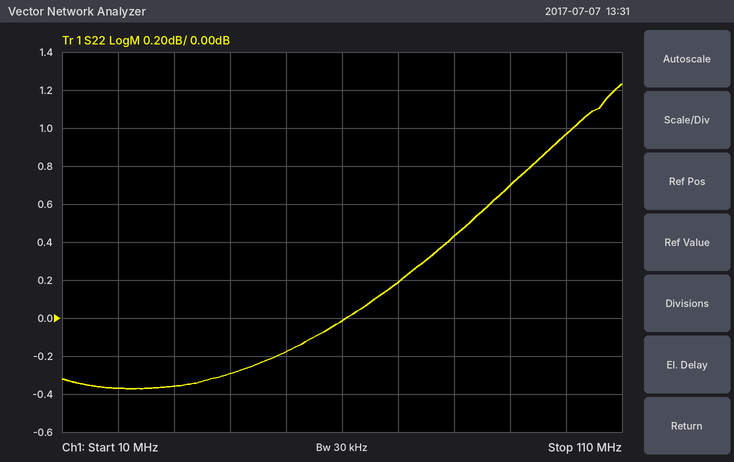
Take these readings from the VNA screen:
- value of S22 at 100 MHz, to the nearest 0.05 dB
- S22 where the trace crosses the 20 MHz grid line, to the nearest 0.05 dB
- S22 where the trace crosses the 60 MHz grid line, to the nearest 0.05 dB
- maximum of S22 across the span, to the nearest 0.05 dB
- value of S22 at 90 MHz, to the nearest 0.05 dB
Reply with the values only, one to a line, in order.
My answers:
0.95 dB
-0.35 dB
0.00 dB
1.25 dB
0.70 dB
